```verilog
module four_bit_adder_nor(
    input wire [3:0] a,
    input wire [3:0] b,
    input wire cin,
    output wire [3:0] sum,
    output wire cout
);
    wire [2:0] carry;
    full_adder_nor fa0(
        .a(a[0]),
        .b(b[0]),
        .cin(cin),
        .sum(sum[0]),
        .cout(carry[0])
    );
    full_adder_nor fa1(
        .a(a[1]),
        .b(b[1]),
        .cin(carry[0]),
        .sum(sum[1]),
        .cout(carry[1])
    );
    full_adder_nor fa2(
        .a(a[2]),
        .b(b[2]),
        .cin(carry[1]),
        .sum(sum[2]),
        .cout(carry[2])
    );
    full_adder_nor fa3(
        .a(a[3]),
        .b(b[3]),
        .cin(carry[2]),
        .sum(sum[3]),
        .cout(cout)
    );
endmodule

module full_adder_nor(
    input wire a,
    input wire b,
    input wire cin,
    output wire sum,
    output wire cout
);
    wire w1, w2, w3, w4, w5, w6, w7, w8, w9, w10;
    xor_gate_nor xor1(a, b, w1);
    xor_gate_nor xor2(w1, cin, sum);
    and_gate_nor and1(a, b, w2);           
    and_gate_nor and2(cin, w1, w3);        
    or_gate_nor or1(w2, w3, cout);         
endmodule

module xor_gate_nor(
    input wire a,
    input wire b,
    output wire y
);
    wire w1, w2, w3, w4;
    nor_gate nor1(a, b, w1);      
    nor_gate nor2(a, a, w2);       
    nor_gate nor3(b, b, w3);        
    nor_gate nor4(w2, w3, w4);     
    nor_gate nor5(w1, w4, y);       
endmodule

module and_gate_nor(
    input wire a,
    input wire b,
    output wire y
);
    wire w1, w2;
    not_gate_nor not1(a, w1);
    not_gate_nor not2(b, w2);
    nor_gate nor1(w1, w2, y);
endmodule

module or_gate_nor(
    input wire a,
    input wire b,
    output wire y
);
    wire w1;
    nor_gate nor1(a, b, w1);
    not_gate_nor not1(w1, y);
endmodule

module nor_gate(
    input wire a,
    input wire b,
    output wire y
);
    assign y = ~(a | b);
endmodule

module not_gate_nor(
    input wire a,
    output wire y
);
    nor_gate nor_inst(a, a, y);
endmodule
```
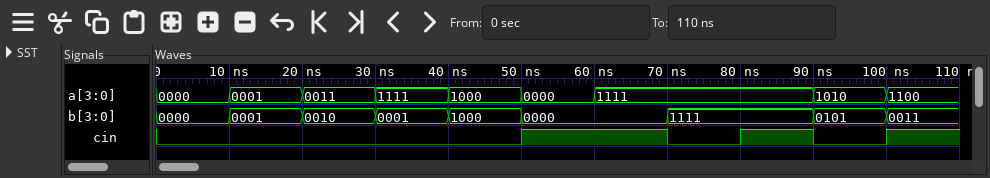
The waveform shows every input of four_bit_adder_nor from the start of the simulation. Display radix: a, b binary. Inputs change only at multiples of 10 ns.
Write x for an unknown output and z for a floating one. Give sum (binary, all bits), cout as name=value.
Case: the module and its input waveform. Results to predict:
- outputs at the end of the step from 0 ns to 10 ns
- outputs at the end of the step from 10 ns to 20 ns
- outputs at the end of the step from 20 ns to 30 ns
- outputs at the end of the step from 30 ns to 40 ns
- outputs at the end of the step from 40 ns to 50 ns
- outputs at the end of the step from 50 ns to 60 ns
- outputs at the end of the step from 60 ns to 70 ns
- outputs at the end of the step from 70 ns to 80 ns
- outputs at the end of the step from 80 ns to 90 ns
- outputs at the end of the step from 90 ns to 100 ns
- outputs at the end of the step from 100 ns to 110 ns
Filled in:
sum=0000, cout=0
sum=0010, cout=0
sum=0101, cout=0
sum=0000, cout=1
sum=0000, cout=1
sum=0001, cout=0
sum=0000, cout=1
sum=1110, cout=1
sum=1111, cout=1
sum=1111, cout=0
sum=0000, cout=1
